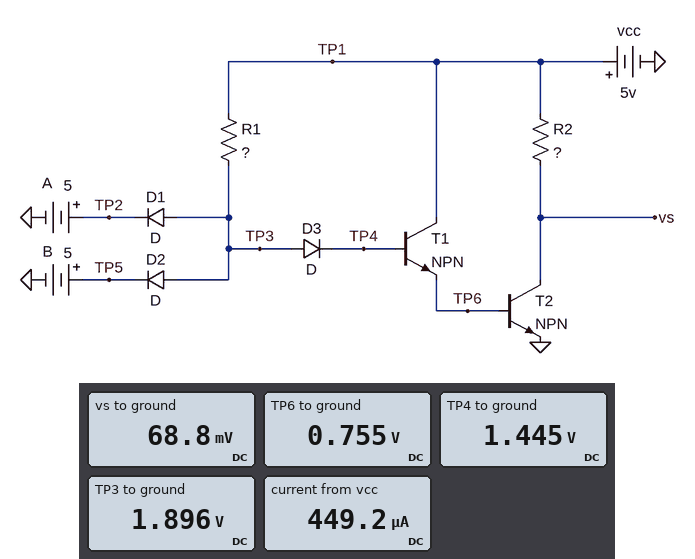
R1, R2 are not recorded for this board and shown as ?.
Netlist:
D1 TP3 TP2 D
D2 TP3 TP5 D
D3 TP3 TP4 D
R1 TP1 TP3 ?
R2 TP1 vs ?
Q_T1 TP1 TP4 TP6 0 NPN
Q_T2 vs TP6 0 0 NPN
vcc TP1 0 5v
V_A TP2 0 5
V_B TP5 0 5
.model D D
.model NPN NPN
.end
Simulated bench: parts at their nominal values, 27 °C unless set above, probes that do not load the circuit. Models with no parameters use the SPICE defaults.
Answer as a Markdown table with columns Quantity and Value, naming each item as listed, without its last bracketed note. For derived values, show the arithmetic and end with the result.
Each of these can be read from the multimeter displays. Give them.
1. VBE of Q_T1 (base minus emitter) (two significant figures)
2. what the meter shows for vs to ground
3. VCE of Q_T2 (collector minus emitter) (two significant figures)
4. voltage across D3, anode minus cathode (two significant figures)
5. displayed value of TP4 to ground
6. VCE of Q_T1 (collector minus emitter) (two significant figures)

| Quantity | Value |
|---|---|
| VBE of Q_T1 (base minus emitter) | 1.445 V - 755 mV = 690 mV |
| what the meter shows for vs to ground | 68.8 mV |
| VCE of Q_T2 (collector minus emitter) | 68.8 mV = 69 mV |
| voltage across D3, anode minus cathode | 1.896 V - 1.445 V = 450 mV |
| displayed value of TP4 to ground | 1.445 V |
| VCE of Q_T1 (collector minus emitter) | 5 V - 755 mV = 4.2 V |
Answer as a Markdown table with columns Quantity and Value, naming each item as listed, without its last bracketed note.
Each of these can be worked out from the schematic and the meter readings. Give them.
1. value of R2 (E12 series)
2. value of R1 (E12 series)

| Quantity | Value |
|---|---|
| value of R2 | 12 kΩ |
| value of R1 | 8.2 MΩ |
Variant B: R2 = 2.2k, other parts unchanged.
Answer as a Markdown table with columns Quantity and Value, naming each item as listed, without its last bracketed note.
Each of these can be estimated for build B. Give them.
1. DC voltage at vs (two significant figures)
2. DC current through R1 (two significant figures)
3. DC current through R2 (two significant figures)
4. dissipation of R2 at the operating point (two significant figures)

| Quantity | Value |
|---|---|
| DC voltage at vs | 130 mV |
| DC current through R1 | 370 nA |
| DC current through R2 | 2.2 mA |
| dissipation of R2 at the operating point | 11 mW |
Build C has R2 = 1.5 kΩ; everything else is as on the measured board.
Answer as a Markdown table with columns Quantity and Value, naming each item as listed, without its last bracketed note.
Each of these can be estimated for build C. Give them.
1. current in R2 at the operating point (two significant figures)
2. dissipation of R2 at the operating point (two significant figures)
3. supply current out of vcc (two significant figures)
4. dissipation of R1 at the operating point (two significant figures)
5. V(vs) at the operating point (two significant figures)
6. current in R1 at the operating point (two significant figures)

| Quantity | Value |
|---|---|
| current in R2 at the operating point | 3.2 mA |
| dissipation of R2 at the operating point | 16 mW |
| supply current out of vcc | 3.3 mA |
| dissipation of R1 at the operating point | 1.1 µW |
| V(vs) at the operating point | 170 mV |
| current in R1 at the operating point | 370 nA |
